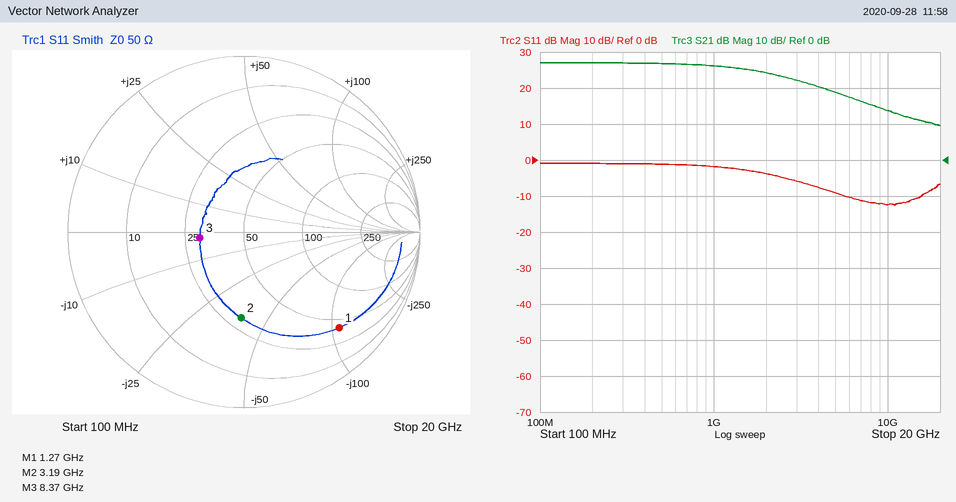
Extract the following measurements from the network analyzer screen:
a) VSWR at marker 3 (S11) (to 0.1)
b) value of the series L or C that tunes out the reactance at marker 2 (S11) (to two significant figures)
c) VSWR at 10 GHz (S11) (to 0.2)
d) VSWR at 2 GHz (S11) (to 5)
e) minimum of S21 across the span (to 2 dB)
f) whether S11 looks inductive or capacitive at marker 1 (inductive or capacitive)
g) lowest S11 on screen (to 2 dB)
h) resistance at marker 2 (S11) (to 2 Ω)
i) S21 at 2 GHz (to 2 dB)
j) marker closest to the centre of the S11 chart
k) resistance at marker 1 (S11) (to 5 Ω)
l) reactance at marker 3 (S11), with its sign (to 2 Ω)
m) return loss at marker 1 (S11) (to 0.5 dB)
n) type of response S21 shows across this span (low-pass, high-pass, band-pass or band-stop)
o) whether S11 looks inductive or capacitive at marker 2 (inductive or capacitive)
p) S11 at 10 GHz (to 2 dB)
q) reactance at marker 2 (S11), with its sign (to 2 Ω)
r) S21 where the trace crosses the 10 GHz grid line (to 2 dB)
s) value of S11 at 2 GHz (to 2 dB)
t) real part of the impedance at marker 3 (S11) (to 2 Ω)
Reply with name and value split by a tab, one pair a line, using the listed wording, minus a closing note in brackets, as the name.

VSWR at marker 3 (S11)	1.7
value of the series L or C that tunes out the reactance at marker 2 (S11)	1.9 nH
VSWR at 10 GHz (S11)	1.6
VSWR at 2 GHz (S11)	5
minimum of S21 across the span	10 dB
whether S11 looks inductive or capacitive at marker 1	capacitive
lowest S11 on screen	-12 dB
resistance at marker 2 (S11)	30 Ω
S21 at 2 GHz	24 dB
marker closest to the centre of the S11 chart	marker 3
resistance at marker 1 (S11)	40 Ω
reactance at marker 3 (S11), with its sign	-2 Ω
return loss at marker 1 (S11)	2.5 dB
type of response S21 shows across this span	low-pass
whether S11 looks inductive or capacitive at marker 2	capacitive
S11 at 10 GHz	-12 dB
reactance at marker 2 (S11), with its sign	-38 Ω
S21 where the trace crosses the 10 GHz grid line	14 dB
value of S11 at 2 GHz	-4 dB
real part of the impedance at marker 3 (S11)	30 Ω
